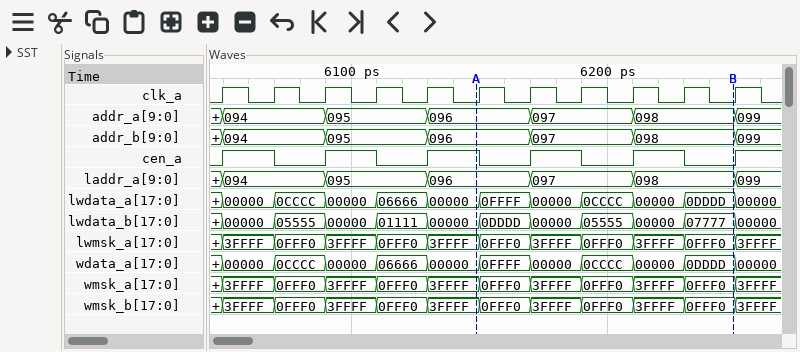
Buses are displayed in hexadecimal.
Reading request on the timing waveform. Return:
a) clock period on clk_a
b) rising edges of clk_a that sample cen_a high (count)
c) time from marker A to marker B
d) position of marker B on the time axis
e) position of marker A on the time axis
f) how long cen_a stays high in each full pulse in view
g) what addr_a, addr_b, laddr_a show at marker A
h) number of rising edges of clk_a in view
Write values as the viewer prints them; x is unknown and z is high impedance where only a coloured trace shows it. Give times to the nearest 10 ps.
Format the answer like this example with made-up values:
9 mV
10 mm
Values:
20 ps
5
100 ps
6250 ps
6150 ps
20 ps, 20 ps, 20 ps, 20 ps, 20 ps
addr_a=096, addr_b=096, laddr_a=096
11
